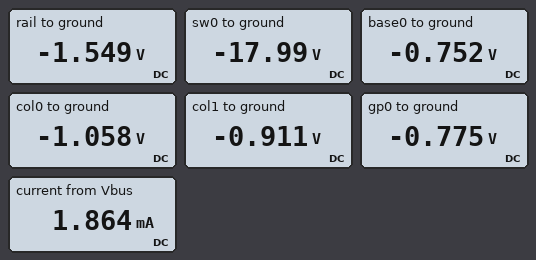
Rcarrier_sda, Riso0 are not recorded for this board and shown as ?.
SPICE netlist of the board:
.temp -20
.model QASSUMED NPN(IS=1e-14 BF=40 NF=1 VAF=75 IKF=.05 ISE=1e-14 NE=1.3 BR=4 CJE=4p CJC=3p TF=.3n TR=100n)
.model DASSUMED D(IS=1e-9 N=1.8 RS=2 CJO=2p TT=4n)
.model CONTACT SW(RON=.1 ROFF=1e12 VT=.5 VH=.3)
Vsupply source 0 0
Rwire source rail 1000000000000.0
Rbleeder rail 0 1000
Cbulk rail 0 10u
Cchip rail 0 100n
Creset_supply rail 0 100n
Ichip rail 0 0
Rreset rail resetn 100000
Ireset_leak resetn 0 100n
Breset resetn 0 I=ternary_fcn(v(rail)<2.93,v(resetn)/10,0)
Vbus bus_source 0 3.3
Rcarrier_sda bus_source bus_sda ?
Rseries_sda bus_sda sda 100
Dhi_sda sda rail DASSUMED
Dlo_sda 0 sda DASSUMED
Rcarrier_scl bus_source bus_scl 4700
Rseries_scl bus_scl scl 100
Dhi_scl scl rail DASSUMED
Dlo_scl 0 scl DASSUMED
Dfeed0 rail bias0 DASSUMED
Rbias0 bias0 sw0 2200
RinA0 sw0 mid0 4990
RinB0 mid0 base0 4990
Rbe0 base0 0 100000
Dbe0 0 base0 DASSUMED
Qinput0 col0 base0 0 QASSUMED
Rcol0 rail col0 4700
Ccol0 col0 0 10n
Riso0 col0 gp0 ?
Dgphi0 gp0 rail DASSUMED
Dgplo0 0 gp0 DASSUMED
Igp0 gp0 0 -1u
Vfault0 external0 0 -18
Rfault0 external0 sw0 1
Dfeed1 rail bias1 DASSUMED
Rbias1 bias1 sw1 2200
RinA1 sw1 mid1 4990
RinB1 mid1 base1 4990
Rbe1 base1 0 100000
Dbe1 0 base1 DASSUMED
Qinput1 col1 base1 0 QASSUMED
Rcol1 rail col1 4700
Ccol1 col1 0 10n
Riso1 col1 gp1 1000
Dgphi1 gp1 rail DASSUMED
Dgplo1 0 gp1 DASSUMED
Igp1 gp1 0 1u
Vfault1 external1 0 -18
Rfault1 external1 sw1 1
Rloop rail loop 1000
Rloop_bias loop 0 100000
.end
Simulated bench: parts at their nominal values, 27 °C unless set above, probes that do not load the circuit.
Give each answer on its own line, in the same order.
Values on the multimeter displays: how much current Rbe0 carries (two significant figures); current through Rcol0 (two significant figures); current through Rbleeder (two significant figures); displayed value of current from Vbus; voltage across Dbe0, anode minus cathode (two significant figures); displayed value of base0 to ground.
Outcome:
7.5 µA
100 µA
1.5 mA
1.864 mA
750 mV
-0.752 V
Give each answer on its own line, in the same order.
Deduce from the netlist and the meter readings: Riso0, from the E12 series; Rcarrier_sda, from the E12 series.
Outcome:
2.7 kΩ
3.9 kΩ
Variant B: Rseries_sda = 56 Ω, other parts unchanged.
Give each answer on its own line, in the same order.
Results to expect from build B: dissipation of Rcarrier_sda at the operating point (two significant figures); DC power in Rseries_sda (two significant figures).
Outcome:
4.1 mW
59 µW
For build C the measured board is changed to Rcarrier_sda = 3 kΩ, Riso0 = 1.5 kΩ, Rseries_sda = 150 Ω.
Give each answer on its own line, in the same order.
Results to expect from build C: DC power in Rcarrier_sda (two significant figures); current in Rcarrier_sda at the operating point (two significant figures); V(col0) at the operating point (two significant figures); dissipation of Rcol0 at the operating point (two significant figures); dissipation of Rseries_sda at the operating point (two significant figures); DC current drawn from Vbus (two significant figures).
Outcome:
5.0 mW
1.3 mA
-960 mV
73 µW
250 µW
2.1 mA
